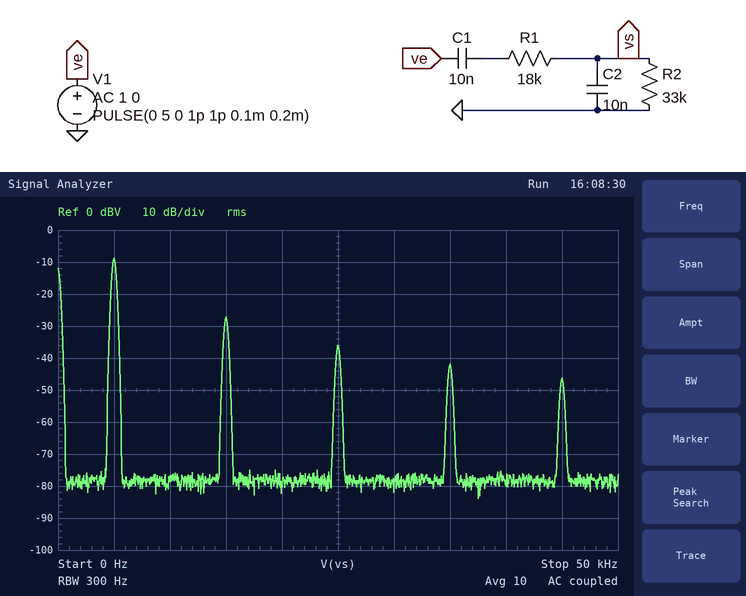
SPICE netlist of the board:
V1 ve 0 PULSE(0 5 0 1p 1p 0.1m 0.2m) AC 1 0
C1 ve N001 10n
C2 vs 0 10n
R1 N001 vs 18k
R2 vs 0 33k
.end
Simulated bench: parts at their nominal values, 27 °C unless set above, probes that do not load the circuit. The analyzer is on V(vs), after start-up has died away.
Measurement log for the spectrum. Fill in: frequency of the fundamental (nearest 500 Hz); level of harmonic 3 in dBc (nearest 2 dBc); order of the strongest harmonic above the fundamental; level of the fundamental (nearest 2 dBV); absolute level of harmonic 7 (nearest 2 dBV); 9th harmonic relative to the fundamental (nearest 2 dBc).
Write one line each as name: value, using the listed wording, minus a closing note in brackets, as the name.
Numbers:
frequency of the fundamental: 5.0 kHz
level of harmonic 3 in dBc: -18 dBc
order of the strongest harmonic above the fundamental: 3
level of the fundamental: -8 dBV
absolute level of harmonic 7: -42 dBV
9th harmonic relative to the fundamental: -38 dBc
